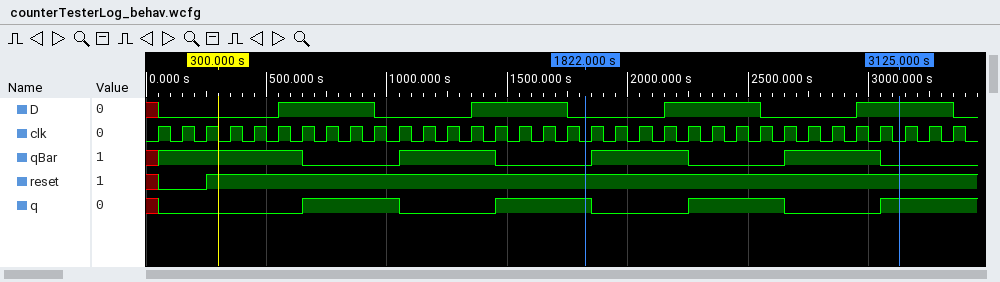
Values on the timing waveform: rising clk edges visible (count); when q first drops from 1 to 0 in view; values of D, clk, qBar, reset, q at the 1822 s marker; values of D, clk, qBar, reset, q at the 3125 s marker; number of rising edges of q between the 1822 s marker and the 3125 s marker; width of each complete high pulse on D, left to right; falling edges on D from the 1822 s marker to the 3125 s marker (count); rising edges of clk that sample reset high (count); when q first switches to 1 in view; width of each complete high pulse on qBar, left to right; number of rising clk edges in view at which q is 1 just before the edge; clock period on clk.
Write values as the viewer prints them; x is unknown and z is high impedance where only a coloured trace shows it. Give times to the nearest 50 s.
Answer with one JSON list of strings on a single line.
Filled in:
["34", "1050 s", "D=0, clk=0, qBar=0, reset=1, q=1", "D=1, clk=0, qBar=0, reset=1, q=1", "2", "400 s, 400 s, 400 s, 400 s", "1", "31", "650 s", "400 s, 400 s, 400 s", "15", "100 s"]
